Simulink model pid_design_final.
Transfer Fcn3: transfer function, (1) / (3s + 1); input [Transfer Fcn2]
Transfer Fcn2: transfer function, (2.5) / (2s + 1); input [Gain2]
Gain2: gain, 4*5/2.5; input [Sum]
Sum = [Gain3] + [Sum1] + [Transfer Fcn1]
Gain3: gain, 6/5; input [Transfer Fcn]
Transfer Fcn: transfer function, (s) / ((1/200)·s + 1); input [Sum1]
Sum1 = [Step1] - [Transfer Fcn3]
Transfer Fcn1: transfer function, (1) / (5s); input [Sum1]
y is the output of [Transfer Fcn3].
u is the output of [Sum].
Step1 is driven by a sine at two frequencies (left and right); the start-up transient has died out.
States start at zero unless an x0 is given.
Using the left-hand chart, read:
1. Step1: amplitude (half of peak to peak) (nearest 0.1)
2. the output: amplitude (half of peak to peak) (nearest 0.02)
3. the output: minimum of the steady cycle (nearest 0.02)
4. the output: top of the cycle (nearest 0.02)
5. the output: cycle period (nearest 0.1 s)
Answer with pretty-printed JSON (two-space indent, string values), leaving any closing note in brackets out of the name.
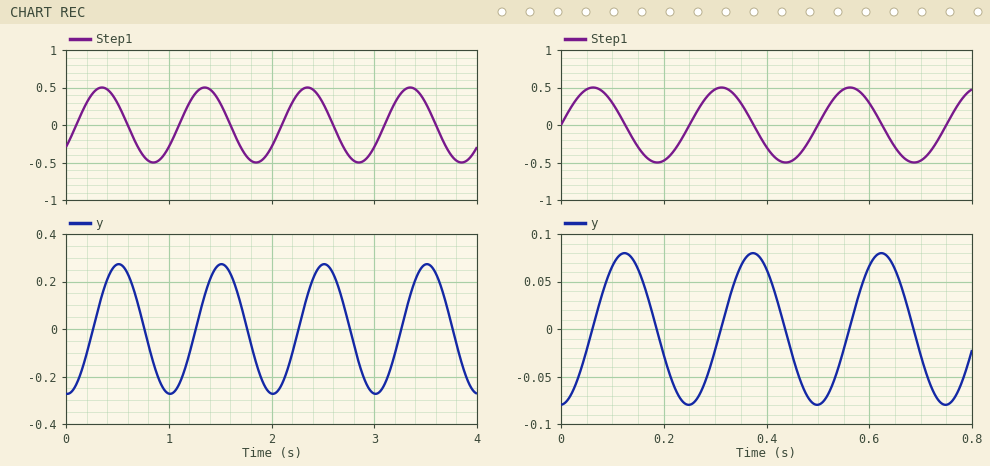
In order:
{
  "Step1: amplitude (half of peak to peak)": "0.5",
  "the output: amplitude (half of peak to peak)": "0.28",
  "the output: minimum of the steady cycle": "-0.28",
  "the output: top of the cycle": "0.28",
  "the output: cycle period": "1.0 s"
}
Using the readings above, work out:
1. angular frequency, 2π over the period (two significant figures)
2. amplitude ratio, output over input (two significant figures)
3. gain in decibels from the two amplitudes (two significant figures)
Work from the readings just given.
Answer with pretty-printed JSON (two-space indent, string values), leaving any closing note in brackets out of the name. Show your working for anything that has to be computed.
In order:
{
  "angular frequency, 2π over the period": "2π / 1 = 6.3 rad/s",
  "amplitude ratio, output over input": "0.28 / 0.5 = 0.56",
  "gain in decibels from the two amplitudes": "20 log10(0.28 / 0.5) = -5.0 dB"
}
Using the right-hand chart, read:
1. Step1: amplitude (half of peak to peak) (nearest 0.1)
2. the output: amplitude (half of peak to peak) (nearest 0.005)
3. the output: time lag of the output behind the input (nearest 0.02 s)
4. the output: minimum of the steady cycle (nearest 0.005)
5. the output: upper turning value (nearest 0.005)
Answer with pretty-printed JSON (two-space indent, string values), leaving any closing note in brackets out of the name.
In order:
{
  "Step1: amplitude (half of peak to peak)": "0.5",
  "the output: amplitude (half of peak to peak)": "0.080",
  "the output: time lag of the output behind the input": "0.06 s",
  "the output: minimum of the steady cycle": "-0.080",
  "the output: upper turning value": "0.080"
}
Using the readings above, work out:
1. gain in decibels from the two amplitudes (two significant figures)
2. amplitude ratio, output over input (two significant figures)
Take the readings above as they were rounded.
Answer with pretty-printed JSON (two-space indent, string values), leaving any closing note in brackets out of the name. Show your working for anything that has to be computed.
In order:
{
  "gain in decibels from the two amplitudes": "20 log10(0.08 / 0.5) = -16 dB",
  "amplitude ratio, output over input": "0.08 / 0.5 = 0.16"
}
